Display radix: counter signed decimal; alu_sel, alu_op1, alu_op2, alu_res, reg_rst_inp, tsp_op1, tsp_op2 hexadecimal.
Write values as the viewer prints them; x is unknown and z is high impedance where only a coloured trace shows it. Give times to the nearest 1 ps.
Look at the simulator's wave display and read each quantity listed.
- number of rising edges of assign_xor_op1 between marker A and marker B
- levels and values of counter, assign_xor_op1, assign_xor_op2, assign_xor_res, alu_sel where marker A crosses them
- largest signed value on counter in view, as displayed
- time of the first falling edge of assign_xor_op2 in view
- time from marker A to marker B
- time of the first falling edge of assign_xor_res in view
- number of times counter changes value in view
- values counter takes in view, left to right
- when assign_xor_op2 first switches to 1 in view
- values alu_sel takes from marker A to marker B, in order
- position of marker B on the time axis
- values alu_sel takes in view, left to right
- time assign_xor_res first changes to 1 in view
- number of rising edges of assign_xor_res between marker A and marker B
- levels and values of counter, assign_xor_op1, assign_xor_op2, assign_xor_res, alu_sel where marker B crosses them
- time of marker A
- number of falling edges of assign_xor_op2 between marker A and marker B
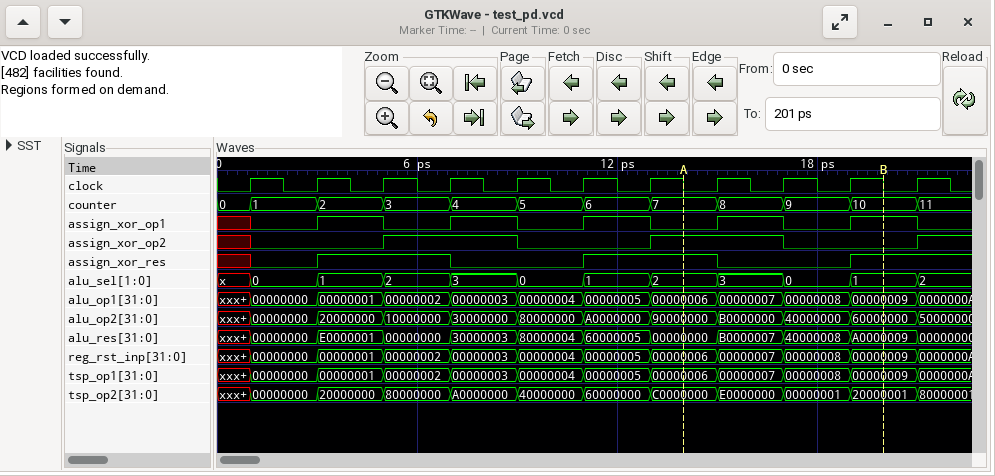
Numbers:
2
counter=7, assign_xor_op1=0, assign_xor_op2=1, assign_xor_res=1, alu_sel=2
11
9 ps
6 ps
7 ps
11
0, 1, 2, 3, 4, 5, 6, 7, 8, 9, 10, 11
5 ps
2, 3, 0, 1
20 ps
x, 0, 1, 2, 3, 0, 1, 2, 3, 0, 1, 2
3 ps
1
counter=10, assign_xor_op1=1, assign_xor_op2=0, assign_xor_res=1, alu_sel=1
14 ps
1
